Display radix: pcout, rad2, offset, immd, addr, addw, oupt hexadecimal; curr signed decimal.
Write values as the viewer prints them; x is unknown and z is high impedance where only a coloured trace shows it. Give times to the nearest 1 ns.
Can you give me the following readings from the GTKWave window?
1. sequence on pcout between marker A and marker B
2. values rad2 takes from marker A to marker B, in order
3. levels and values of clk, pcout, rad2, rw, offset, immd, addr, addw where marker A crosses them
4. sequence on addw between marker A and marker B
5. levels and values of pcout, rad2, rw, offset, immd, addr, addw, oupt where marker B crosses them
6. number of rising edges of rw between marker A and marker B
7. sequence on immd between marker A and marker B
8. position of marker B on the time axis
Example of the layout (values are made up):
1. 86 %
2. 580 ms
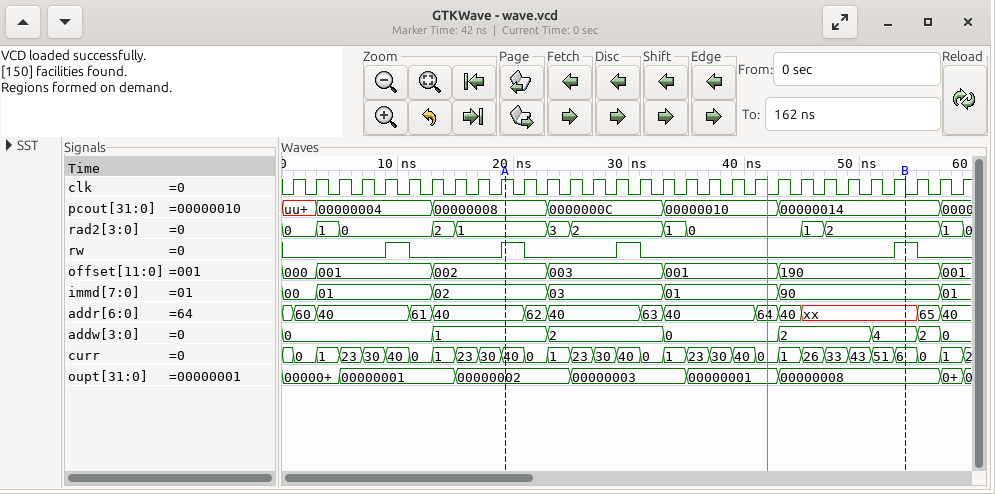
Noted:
1. 00000008, 0000000C, 00000010, 00000014
2. 1, 3, 2, 1, 0, 1, 2
3. clk=1, pcout=00000008, rad2=1, rw=1, offset=002, immd=02, addr=40, addw=1
4. 1, 2, 0, 2, 4
5. pcout=00000014, rad2=2, rw=1, offset=190, immd=90, addr=xx, addw=4, oupt=00000008
6. 2
7. 02, 03, 01, 90
8. 54 ns
